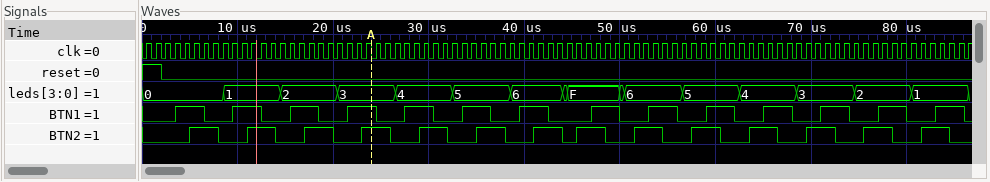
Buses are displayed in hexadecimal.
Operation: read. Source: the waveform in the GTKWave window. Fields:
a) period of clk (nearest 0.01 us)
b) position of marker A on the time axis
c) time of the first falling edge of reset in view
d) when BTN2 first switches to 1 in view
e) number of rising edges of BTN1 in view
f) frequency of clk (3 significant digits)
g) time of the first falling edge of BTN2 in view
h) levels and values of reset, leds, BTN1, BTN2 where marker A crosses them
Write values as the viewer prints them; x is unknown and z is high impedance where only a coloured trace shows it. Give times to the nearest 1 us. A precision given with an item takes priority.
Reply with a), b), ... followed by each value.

a) 1 us
b) 24 us
c) 2 us
d) 5 us
e) 14
f) 1.00 MHz
g) 8 us
h) reset=0, leds=3, BTN1=1, BTN2=1
